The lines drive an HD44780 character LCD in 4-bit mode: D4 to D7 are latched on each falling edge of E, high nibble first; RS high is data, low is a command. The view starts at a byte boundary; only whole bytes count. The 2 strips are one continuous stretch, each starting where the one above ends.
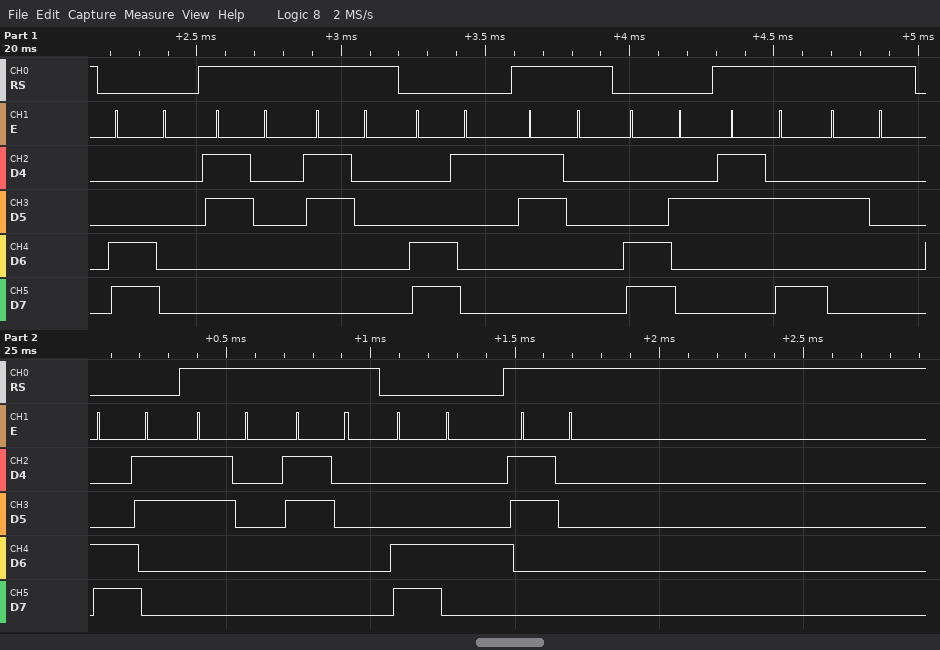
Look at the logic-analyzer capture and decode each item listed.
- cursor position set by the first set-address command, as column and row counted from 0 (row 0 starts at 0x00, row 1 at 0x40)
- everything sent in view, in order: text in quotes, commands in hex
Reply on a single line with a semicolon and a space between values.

column 0, row 1; 0xC0 "00" 0xC1 "0" 0xC2 ": " 0xC3 "00" 0xC4 "0"
